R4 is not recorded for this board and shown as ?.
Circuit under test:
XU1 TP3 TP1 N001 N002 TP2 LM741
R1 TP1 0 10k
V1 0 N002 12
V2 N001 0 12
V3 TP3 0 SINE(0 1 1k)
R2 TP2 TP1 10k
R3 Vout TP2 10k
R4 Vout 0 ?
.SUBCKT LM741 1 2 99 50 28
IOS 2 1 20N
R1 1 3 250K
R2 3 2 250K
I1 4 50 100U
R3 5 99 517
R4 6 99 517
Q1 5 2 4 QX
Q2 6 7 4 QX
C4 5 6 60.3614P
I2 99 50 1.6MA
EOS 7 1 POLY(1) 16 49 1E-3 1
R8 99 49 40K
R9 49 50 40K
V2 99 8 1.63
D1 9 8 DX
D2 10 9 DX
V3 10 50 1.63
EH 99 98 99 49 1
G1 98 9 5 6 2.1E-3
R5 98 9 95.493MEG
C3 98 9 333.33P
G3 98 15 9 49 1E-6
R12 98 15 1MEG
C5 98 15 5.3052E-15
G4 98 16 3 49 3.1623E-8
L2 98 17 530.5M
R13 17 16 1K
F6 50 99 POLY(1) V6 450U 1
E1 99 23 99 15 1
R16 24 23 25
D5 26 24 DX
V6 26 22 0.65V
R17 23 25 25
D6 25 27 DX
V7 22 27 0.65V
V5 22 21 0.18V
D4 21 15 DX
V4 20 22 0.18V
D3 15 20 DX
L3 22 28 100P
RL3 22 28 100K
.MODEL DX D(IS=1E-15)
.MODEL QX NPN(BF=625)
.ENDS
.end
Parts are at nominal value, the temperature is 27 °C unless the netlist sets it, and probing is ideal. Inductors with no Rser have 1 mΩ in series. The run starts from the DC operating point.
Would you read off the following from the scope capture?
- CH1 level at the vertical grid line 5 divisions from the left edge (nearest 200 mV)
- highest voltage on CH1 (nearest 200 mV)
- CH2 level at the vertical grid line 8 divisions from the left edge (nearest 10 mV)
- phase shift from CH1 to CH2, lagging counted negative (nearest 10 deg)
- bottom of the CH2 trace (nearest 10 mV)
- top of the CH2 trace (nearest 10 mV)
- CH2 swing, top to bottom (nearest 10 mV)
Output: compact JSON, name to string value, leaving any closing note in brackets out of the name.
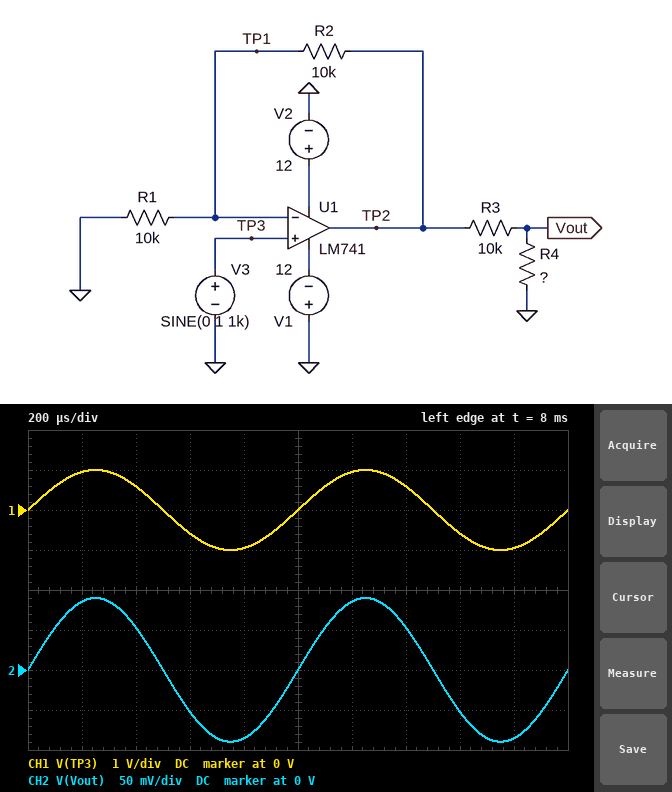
{"CH1 level at the vertical grid line 5 divisions from the left edge": "0 V", "highest voltage on CH1": "1.0 V", "CH2 level at the vertical grid line 8 divisions from the left edge": "-50 mV", "phase shift from CH1 to CH2, lagging counted negative": "0 deg", "bottom of the CH2 trace": "-90 mV", "top of the CH2 trace": "90 mV", "CH2 swing, top to bottom": "180 mV"}
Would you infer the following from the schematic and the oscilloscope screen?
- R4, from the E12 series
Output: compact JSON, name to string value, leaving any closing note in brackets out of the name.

{"R4, from the E12 series": "470 Ω"}
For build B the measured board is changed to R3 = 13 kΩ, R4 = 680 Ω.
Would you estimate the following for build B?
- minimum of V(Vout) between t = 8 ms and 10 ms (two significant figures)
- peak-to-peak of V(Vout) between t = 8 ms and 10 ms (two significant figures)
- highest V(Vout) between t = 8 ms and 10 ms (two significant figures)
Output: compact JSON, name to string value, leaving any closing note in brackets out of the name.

{"minimum of V(Vout) between t = 8 ms and 10 ms": "-99 mV", "peak-to-peak of V(Vout) between t = 8 ms and 10 ms": "200 mV", "highest V(Vout) between t = 8 ms and 10 ms": "100 mV"}
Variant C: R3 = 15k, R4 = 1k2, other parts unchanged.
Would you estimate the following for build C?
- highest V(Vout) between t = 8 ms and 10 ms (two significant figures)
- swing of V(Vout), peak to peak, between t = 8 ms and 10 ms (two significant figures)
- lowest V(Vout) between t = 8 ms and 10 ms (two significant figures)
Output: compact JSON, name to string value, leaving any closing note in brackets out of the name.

{"highest V(Vout) between t = 8 ms and 10 ms": "150 mV", "swing of V(Vout), peak to peak, between t = 8 ms and 10 ms": "300 mV", "lowest V(Vout) between t = 8 ms and 10 ms": "-150 mV"}
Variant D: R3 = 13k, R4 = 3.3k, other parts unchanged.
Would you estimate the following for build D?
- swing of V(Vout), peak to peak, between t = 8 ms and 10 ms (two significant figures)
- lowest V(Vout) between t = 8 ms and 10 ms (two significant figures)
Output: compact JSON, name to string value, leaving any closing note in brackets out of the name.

{"swing of V(Vout), peak to peak, between t = 8 ms and 10 ms": "810 mV", "lowest V(Vout) between t = 8 ms and 10 ms": "-400 mV"}
